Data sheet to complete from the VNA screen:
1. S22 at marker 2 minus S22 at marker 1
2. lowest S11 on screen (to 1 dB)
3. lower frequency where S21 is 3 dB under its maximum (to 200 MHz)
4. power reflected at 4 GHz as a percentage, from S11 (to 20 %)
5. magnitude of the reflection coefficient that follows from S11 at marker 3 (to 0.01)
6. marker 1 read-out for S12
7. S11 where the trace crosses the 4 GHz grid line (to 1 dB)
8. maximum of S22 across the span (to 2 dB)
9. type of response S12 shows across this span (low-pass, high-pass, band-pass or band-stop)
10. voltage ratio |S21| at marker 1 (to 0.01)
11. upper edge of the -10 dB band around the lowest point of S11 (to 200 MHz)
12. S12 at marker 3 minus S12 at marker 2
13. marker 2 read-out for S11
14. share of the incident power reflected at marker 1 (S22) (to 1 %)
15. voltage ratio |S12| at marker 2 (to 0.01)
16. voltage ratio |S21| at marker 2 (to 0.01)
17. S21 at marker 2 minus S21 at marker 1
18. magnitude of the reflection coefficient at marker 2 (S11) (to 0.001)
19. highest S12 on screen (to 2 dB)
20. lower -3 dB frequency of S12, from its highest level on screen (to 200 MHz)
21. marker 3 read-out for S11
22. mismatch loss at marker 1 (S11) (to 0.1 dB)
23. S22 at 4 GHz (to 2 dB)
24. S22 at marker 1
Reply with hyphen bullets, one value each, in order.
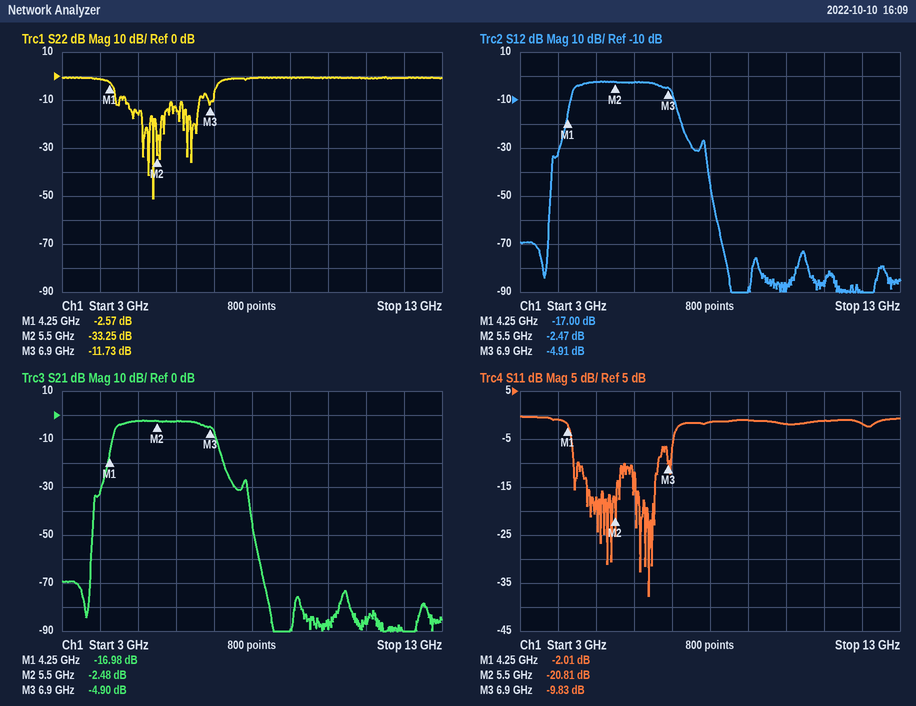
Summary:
- -30.68 dB
- -38 dB
- 4.4 GHz
- 80 %
- 0.32
- -17.00 dB
- -1 dB
- 0 dB
- band-pass
- 0.14
- 6.6 GHz
- -2.44 dB
- -20.81 dB
- 55 %
- 0.75
- 0.75
- 14.50 dB
- 0.091
- -2 dB
- 4.4 GHz
- -9.83 dB
- 4.3 dB
- -2 dB
- -2.57 dB
